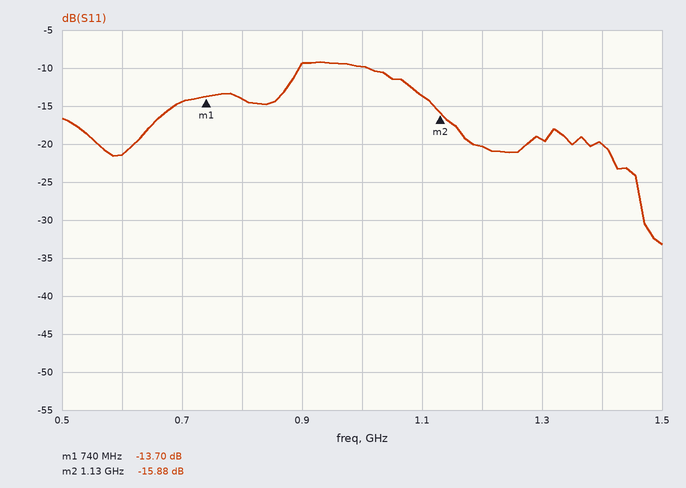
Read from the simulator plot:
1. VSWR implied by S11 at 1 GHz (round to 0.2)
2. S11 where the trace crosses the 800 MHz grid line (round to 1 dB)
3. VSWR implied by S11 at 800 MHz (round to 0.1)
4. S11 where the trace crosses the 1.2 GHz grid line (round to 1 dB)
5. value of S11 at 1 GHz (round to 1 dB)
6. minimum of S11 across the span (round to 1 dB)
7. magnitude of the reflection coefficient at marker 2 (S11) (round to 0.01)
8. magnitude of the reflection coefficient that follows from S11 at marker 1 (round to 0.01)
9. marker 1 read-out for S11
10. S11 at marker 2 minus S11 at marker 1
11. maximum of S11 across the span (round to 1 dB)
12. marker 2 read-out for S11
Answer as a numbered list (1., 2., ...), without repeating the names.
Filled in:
1. 2.0
2. -14 dB
3. 1.5
4. -20 dB
5. -10 dB
6. -33 dB
7. 0.16
8. 0.21
9. -13.70 dB
10. -2.18 dB
11. -9 dB
12. -15.88 dB
